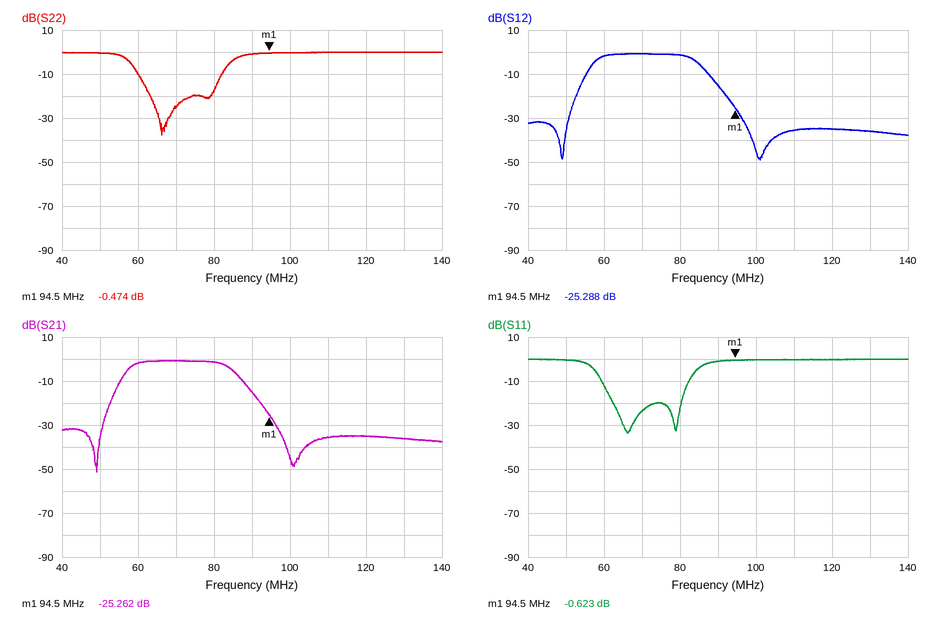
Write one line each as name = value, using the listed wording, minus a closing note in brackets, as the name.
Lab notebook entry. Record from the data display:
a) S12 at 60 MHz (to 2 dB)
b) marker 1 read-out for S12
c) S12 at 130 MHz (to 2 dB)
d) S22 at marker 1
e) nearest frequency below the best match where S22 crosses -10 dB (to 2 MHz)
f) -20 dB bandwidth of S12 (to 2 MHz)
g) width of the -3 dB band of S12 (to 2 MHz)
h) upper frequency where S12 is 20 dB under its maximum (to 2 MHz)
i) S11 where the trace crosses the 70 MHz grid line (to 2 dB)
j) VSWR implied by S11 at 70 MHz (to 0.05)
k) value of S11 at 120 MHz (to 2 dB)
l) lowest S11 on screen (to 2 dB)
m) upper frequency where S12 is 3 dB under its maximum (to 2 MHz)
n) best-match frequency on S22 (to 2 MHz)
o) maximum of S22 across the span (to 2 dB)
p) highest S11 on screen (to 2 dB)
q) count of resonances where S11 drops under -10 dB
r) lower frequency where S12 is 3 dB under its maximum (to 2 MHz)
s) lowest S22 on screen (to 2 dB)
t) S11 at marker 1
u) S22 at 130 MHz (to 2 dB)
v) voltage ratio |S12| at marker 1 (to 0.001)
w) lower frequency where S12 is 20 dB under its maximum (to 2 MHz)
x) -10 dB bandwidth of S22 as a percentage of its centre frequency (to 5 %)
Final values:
S12 at 60 MHz = -2 dB
marker 1 read-out for S12 = -25.288 dB
S12 at 130 MHz = -36 dB
S22 at marker 1 = -0.474 dB
nearest frequency below the best match where S22 crosses -10 dB = 60 MHz
-20 dB bandwidth of S12 = 40 MHz
width of the -3 dB band of S12 = 26 MHz
upper frequency where S12 is 20 dB under its maximum = 92 MHz
S11 where the trace crosses the 70 MHz grid line = -24 dB
VSWR implied by S11 at 70 MHz = 1.15
value of S11 at 120 MHz = 0 dB
lowest S11 on screen = -34 dB
upper frequency where S12 is 3 dB under its maximum = 84 MHz
best-match frequency on S22 = 66 MHz
maximum of S22 across the span = 0 dB
highest S11 on screen = 0 dB
count of resonances where S11 drops under -10 dB = 2
lower frequency where S12 is 3 dB under its maximum = 58 MHz
lowest S22 on screen = -38 dB
S11 at marker 1 = -0.623 dB
S22 at 130 MHz = 0 dB
voltage ratio |S12| at marker 1 = 0.054
lower frequency where S12 is 20 dB under its maximum = 52 MHz
-10 dB bandwidth of S22 as a percentage of its centre frequency = 30 %
